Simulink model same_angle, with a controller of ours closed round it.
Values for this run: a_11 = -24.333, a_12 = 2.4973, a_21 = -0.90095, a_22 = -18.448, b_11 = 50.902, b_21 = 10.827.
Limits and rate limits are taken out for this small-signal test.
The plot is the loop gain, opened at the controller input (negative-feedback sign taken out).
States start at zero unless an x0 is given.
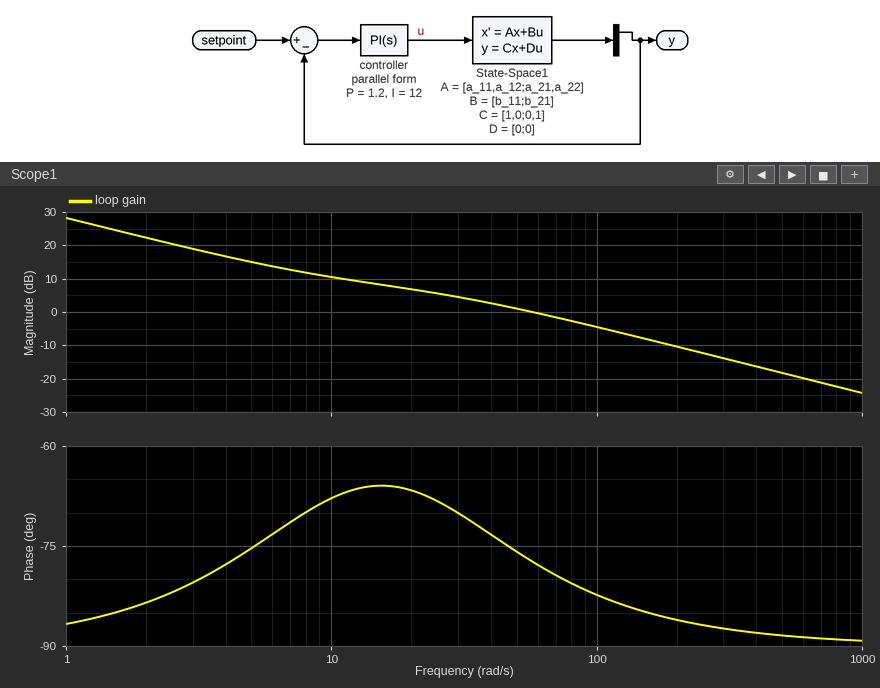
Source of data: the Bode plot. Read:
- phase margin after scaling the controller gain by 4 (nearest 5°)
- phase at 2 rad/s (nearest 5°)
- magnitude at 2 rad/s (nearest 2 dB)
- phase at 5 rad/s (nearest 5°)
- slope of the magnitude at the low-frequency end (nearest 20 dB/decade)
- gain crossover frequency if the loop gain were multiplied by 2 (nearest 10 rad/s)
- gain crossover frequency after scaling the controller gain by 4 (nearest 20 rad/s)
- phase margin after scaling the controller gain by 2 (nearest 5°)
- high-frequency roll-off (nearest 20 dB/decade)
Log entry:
95°
-85°
22 dB
-75°
-20 dB/decade
120 rad/s
240 rad/s
95°
-20 dB/decade
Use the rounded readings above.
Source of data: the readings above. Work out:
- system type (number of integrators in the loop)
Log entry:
1
